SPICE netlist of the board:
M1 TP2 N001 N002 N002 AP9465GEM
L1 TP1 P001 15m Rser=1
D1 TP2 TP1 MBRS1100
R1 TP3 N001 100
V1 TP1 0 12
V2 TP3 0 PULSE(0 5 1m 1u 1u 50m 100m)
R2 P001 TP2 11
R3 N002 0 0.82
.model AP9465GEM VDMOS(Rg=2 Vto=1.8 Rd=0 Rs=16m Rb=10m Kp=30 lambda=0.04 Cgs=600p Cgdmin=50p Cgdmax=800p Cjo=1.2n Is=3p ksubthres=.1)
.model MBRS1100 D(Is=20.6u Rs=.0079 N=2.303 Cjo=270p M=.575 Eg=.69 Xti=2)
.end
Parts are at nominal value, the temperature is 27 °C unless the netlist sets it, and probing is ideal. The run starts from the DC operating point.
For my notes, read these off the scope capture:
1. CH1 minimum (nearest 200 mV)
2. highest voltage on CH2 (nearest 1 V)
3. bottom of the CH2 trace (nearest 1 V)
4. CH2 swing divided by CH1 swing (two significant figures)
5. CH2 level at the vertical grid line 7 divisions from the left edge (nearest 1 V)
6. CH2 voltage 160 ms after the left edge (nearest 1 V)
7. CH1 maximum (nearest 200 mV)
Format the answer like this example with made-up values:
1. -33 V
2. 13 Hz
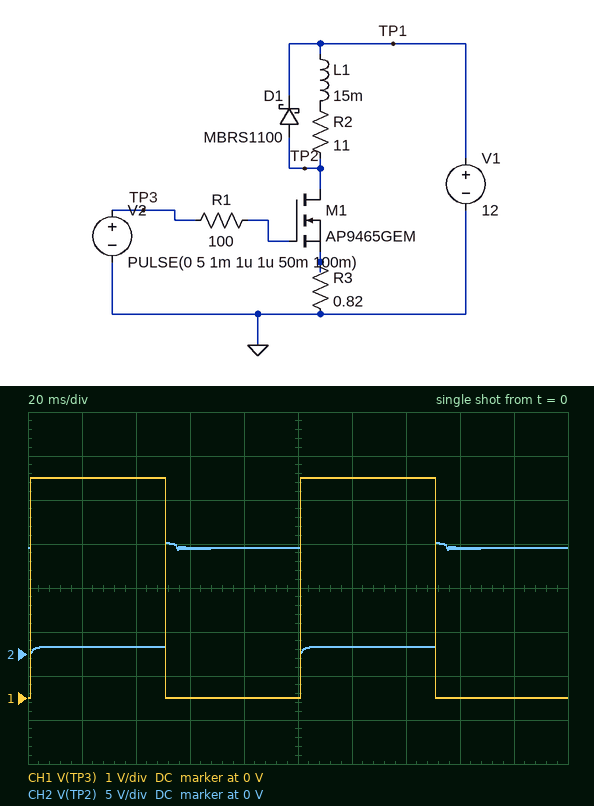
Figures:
1. 0 V
2. 13 V
3. 0 V
4. 2.5
5. 1 V
6. 12 V
7. 5.0 V
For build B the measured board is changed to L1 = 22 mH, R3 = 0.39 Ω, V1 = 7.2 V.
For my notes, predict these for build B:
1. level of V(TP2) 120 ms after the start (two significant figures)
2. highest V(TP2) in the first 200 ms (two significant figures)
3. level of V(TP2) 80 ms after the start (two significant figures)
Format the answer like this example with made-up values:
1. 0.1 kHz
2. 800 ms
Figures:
1. 240 mV
2. 7.8 V
3. 7.2 V
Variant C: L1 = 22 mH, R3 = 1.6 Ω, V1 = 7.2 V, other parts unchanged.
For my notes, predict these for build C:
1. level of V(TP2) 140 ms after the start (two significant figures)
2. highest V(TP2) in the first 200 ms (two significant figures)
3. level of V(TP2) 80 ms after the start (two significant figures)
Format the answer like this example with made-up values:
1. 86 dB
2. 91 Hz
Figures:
1. 860 mV
2. 7.8 V
3. 7.2 V
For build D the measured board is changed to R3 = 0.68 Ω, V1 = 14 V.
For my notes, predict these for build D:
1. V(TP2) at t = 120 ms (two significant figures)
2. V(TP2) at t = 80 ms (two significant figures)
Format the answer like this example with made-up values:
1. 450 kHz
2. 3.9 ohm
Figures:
1. 780 mV
2. 14 V
